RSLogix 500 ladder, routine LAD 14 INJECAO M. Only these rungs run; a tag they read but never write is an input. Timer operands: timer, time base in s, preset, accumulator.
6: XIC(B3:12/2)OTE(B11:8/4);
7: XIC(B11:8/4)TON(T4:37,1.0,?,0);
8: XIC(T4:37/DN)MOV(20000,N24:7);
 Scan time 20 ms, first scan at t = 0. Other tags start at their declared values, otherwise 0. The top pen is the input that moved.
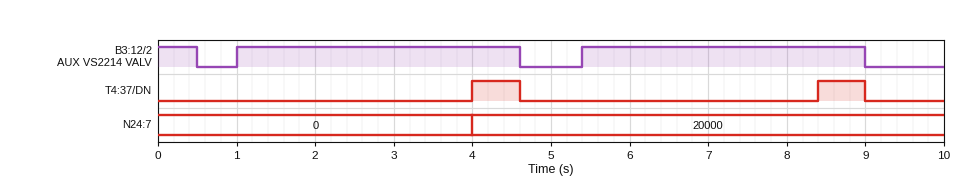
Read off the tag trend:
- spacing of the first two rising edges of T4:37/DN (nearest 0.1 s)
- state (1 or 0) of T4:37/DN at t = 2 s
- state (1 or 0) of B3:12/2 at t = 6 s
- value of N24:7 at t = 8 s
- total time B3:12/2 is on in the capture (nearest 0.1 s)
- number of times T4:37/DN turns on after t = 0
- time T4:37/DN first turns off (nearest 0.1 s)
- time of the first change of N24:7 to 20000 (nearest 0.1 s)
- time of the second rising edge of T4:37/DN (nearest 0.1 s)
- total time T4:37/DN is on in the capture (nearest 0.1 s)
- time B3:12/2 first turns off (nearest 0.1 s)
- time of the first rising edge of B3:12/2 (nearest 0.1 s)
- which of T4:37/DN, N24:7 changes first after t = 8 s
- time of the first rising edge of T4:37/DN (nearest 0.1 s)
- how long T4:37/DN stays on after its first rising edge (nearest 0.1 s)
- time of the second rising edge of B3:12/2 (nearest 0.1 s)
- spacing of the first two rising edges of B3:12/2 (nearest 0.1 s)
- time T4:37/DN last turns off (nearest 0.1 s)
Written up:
4.4 s
0
1
20000
7.7 s
2
4.6 s
4.0 s
8.4 s
1.2 s
0.5 s
1.0 s
T4:37/DN
4.0 s
0.6 s
5.4 s
4.4 s
9.0 s
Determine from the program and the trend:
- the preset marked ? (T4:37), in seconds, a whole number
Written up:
3 s
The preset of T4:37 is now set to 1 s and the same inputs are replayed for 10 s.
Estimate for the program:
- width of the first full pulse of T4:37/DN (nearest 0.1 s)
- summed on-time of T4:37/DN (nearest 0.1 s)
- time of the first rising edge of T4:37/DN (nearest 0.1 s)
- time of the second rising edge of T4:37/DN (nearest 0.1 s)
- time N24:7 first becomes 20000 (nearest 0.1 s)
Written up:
2.6 s
5.2 s
2.0 s
6.4 s
2.0 s
